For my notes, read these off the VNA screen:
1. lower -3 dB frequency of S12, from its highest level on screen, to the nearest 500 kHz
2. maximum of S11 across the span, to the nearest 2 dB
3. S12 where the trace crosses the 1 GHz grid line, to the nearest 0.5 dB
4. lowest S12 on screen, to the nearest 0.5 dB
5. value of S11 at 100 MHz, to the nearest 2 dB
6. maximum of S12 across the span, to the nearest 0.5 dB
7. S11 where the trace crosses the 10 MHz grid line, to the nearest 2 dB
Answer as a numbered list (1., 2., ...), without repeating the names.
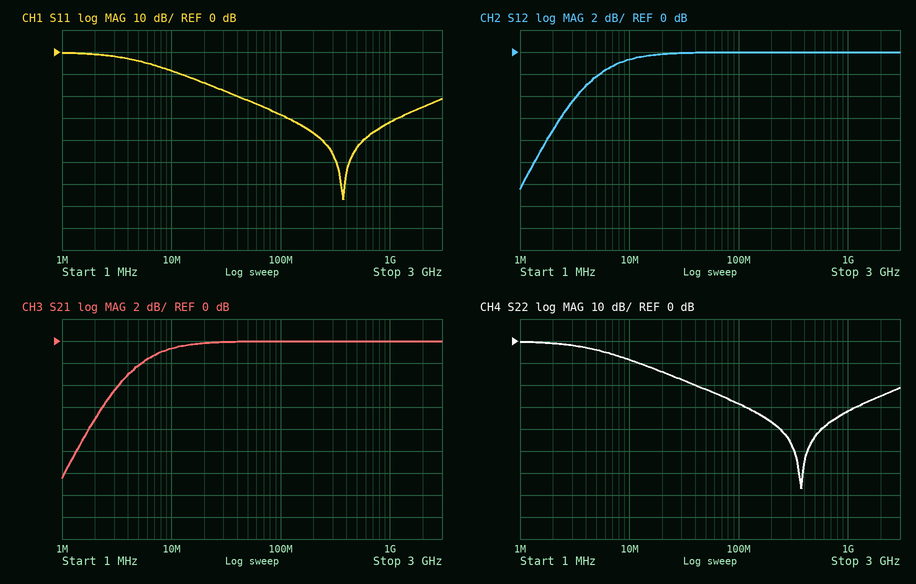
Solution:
1. 4.0 MHz
2. 0 dB
3. 0.0 dB
4. -12.5 dB
5. -28 dB
6. 0.0 dB
7. -8 dB
